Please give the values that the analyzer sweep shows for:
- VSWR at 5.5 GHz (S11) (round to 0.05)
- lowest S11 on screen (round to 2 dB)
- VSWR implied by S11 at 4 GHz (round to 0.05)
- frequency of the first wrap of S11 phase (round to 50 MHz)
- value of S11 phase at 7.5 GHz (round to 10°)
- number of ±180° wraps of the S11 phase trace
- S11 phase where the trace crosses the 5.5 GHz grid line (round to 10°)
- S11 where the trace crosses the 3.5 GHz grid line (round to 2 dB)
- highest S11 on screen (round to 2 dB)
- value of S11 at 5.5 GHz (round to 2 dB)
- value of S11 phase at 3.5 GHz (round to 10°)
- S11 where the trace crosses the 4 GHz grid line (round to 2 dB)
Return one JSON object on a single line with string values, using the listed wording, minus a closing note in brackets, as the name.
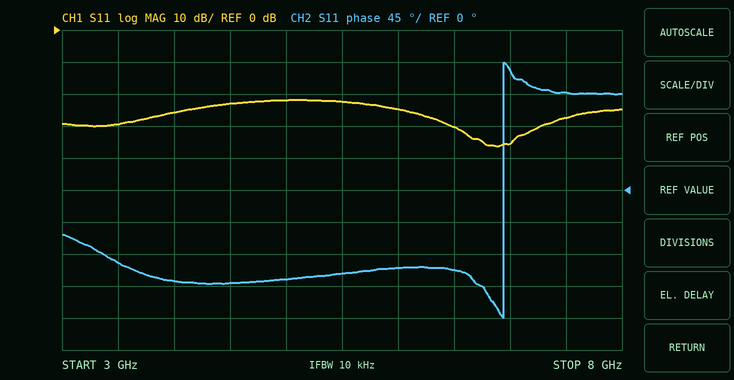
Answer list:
{"VSWR at 5.5 GHz (S11)": "1.15", "lowest S11 on screen": "-36 dB", "VSWR implied by S11 at 4 GHz": "1.10", "frequency of the first wrap of S11 phase": "6.95 GHz", "value of S11 phase at 7.5 GHz": "140°", "number of ±180° wraps of the S11 phase trace": "1", "S11 phase where the trace crosses the 5.5 GHz grid line": "-120°", "S11 where the trace crosses the 3.5 GHz grid line": "-30 dB", "highest S11 on screen": "-22 dB", "value of S11 at 5.5 GHz": "-22 dB", "value of S11 phase at 3.5 GHz": "-100°", "S11 where the trace crosses the 4 GHz grid line": "-26 dB"}
